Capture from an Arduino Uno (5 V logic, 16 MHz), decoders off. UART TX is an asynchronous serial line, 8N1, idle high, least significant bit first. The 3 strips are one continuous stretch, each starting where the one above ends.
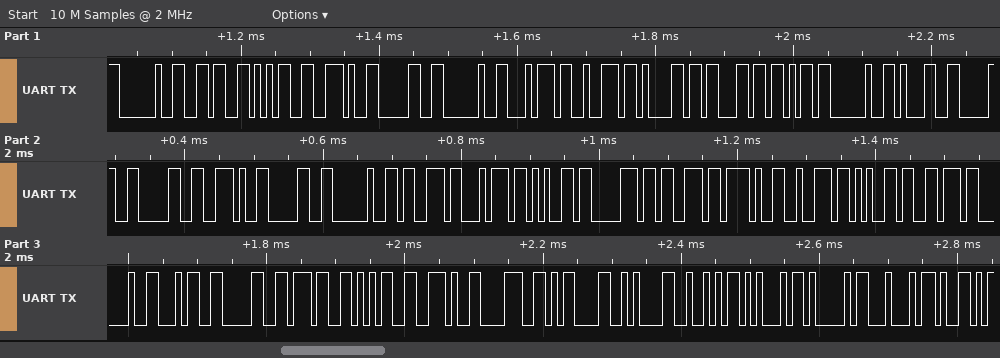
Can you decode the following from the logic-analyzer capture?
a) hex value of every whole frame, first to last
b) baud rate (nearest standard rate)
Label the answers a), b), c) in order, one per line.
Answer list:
a) 20 36 35 2E 30 20 74 72 61 63 6B 20 31 30 30 2E 30 20 73 74 65 70 73 2F 72 65 76 20 34 30 37 35 2E 38 0D 0A 52 45 41 44 59
b) 115200 baud
